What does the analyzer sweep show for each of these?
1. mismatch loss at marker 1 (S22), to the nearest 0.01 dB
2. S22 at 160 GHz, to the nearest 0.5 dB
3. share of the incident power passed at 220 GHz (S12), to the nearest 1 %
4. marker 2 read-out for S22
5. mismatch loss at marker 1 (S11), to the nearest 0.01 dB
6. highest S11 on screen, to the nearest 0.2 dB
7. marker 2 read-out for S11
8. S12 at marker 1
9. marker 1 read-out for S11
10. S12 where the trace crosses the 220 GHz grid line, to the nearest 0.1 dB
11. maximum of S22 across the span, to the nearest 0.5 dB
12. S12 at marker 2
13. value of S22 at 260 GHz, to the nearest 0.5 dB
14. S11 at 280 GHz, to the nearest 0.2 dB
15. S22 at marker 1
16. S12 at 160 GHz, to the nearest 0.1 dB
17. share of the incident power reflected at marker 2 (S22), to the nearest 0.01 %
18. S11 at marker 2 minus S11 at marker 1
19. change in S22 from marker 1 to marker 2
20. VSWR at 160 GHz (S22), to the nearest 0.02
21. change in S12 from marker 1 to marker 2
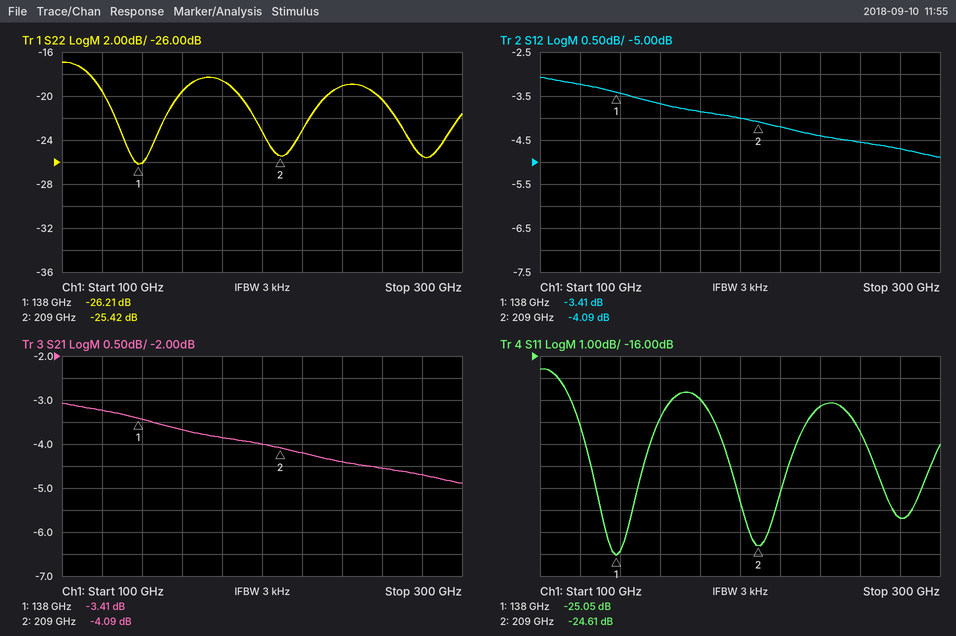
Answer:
0.01 dB
-19.5 dB
38 %
-25.42 dB
0.01 dB
-16.6 dB
-24.61 dB
-3.41 dB
-25.05 dB
-4.2 dB
-17.0 dB
-4.09 dB
-20.5 dB
-23.4 dB
-26.21 dB
-3.7 dB
0.29 %
0.44 dB
0.79 dB
1.24
-0.68 dB
